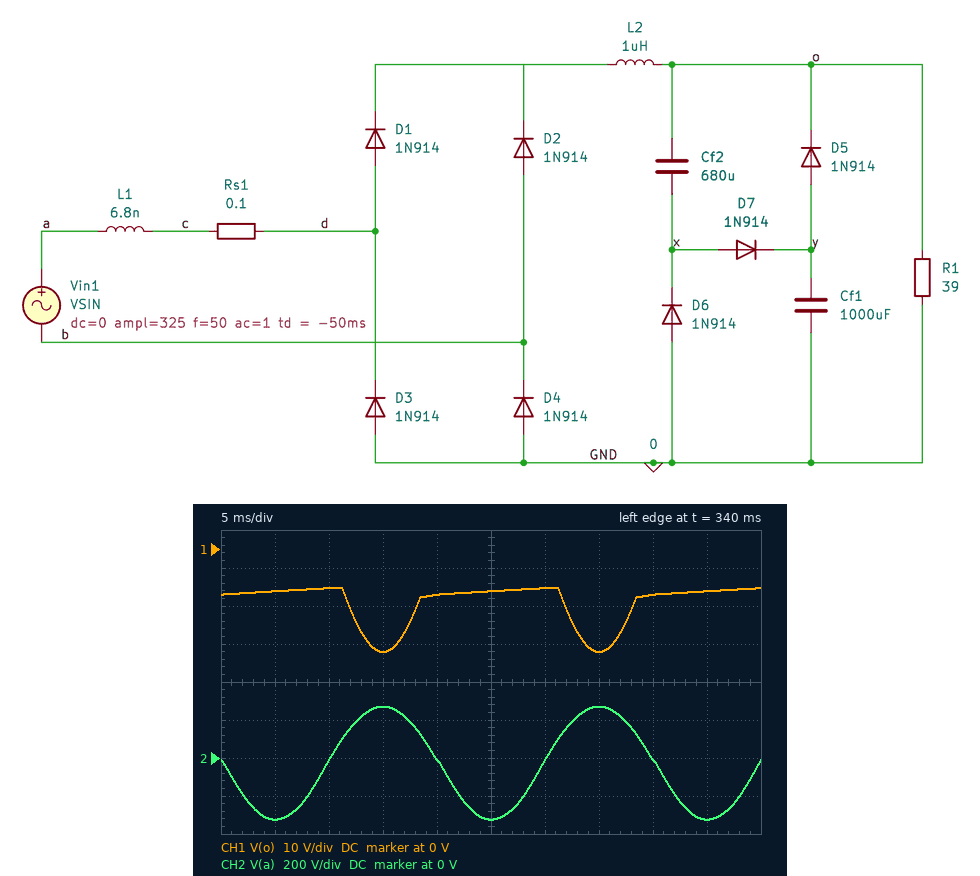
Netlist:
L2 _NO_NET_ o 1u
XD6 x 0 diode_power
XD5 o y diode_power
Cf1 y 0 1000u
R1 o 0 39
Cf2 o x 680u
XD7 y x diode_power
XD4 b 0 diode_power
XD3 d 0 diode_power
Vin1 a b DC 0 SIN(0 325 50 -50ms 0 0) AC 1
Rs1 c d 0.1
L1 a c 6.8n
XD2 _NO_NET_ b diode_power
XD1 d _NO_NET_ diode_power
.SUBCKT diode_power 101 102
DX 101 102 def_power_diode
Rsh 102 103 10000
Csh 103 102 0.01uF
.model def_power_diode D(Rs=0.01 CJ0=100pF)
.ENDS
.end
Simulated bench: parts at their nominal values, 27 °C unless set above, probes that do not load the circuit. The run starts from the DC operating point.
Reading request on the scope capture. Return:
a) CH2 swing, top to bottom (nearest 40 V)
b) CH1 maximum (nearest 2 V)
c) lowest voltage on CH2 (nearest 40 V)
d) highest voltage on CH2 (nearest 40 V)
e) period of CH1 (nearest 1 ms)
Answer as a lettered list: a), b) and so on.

a) 600 V
b) -10 V
c) -320 V
d) 280 V
e) 20 ms
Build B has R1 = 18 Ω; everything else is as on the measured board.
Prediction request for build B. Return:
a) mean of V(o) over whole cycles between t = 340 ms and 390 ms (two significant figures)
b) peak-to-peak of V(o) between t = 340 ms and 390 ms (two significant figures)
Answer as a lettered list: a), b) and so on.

a) -14 V
b) 19 V
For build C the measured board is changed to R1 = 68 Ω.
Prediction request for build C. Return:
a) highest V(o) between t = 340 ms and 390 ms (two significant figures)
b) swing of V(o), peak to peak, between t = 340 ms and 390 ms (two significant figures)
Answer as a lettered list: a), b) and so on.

a) -11 V
b) 16 V
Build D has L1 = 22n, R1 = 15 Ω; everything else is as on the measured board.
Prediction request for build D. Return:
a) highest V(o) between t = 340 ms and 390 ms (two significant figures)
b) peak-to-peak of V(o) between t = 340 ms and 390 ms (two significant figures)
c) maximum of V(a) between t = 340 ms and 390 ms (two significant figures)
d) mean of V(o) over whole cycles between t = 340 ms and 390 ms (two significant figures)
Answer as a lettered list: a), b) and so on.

a) -7.4 V
b) 20 V
c) 270 V
d) -14 V
